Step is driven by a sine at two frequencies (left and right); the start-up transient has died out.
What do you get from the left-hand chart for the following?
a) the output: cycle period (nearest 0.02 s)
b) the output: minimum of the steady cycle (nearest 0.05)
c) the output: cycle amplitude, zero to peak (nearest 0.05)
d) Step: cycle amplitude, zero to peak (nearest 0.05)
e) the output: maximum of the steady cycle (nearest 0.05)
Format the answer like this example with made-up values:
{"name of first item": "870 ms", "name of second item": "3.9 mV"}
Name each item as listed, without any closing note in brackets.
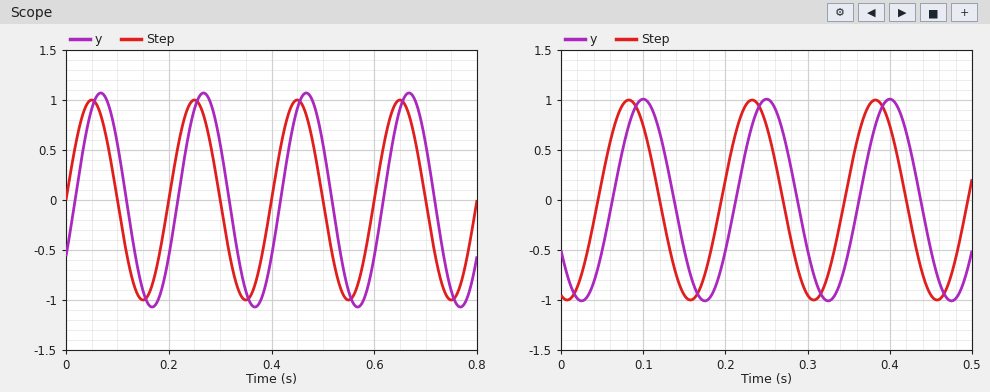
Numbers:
{"the output: cycle period": "0.20 s", "the output: minimum of the steady cycle": "-1.05", "the output: cycle amplitude, zero to peak": "1.05", "Step: cycle amplitude, zero to peak": "1.00", "the output: maximum of the steady cycle": "1.05"}
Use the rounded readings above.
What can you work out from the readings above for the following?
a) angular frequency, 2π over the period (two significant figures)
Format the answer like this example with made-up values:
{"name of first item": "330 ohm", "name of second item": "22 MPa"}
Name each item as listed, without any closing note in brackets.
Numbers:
{"angular frequency, 2π over the period": "31 rad/s"}
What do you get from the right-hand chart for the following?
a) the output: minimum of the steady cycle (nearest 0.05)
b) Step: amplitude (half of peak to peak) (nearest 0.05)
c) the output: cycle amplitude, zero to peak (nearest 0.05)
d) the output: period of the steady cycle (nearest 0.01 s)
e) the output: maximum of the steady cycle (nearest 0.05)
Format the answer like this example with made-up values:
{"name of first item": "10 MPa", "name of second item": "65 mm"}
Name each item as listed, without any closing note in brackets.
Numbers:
{"the output: minimum of the steady cycle": "-1.00", "Step: amplitude (half of peak to peak)": "1.00", "the output: cycle amplitude, zero to peak": "1.00", "the output: period of the steady cycle": "0.15 s", "the output: maximum of the steady cycle": "1.00"}
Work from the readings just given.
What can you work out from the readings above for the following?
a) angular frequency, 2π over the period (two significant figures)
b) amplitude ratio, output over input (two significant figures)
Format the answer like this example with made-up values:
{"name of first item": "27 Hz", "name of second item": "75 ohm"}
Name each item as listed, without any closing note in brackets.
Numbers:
{"angular frequency, 2π over the period": "42 rad/s", "amplitude ratio, output over input": "1.0"}
